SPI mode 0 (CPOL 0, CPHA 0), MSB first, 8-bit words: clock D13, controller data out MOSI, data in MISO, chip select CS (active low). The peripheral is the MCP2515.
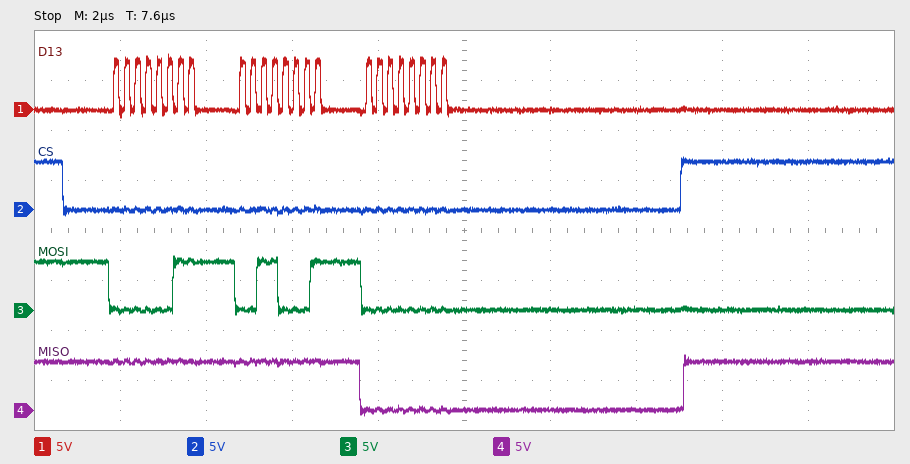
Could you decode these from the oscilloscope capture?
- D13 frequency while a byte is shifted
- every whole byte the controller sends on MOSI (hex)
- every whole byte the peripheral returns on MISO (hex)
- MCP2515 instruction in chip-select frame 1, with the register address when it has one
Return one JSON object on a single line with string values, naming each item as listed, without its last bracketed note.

{"D13 frequency while a byte is shifted": "4 MHz", "every whole byte the controller sends on MOSI": "0x03 0x31 0x00", "every whole byte the peripheral returns on MISO": "0xFF 0xFF 0x00", "MCP2515 instruction in chip-select frame 1, with the register address when it has one": "READ 0x31"}
